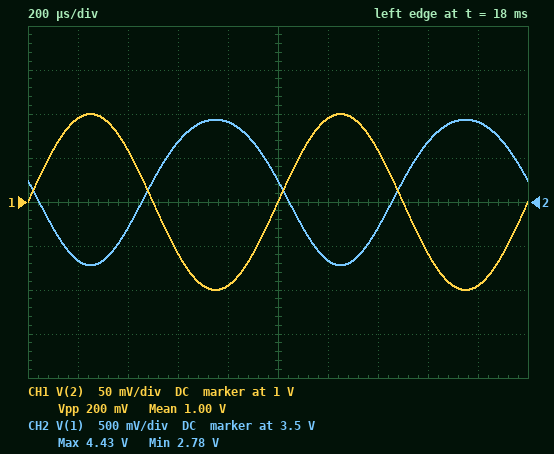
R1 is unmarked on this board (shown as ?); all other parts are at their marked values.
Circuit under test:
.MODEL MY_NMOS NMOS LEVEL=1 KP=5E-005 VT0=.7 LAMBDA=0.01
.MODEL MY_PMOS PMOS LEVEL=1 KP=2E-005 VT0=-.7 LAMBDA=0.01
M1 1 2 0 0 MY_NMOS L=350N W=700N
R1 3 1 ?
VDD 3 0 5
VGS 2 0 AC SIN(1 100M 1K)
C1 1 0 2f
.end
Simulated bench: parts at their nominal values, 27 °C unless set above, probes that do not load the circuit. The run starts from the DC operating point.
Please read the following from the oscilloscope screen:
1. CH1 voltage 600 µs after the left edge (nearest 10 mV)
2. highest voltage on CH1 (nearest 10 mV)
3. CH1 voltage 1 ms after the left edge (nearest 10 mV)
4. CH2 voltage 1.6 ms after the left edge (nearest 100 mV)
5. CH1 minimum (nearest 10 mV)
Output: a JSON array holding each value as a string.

["940 mV", "1.10 V", "1.00 V", "4.2 V", "900 mV"]
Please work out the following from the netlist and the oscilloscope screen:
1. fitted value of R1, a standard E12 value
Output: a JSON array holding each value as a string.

["270 kΩ"]
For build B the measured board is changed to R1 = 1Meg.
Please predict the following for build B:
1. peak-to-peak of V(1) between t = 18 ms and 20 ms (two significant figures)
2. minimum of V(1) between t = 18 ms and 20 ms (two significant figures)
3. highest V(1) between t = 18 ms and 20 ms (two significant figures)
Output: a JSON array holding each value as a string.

["2.8 V", "150 mV", "2.9 V"]
